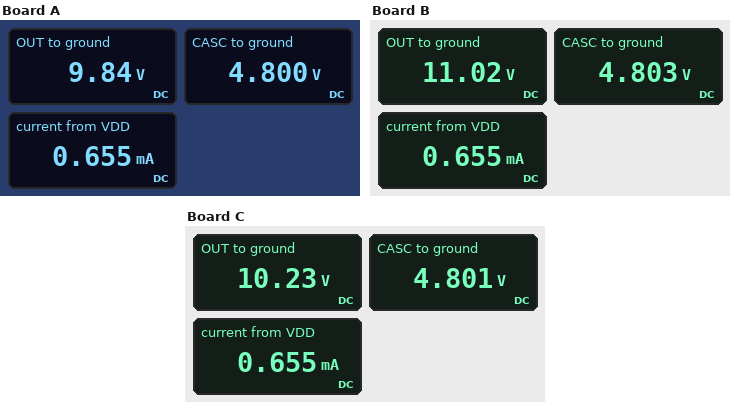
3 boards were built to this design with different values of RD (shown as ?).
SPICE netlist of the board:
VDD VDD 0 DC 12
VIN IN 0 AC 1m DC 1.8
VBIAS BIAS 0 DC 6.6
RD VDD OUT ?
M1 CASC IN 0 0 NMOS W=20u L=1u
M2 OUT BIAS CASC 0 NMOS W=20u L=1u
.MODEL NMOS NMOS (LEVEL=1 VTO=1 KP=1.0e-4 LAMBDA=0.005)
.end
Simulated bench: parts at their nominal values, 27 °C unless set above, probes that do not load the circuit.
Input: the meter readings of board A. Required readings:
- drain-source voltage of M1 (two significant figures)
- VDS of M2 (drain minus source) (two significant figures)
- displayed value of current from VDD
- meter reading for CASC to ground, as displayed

4.8 V
5.0 V
0.655 mA
4.800 V
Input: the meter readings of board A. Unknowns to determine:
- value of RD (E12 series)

3.3 kΩ
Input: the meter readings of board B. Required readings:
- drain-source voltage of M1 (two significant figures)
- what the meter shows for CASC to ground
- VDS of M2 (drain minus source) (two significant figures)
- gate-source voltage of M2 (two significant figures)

4.8 V
4.803 V
6.2 V
1.8 V
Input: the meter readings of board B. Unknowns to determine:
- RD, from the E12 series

1.5 kΩ
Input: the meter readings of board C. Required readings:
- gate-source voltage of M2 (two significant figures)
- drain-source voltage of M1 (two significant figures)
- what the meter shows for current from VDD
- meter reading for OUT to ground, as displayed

1.8 V
4.8 V
0.655 mA
10.23 V
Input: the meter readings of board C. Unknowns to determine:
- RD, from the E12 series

2.7 kΩ
